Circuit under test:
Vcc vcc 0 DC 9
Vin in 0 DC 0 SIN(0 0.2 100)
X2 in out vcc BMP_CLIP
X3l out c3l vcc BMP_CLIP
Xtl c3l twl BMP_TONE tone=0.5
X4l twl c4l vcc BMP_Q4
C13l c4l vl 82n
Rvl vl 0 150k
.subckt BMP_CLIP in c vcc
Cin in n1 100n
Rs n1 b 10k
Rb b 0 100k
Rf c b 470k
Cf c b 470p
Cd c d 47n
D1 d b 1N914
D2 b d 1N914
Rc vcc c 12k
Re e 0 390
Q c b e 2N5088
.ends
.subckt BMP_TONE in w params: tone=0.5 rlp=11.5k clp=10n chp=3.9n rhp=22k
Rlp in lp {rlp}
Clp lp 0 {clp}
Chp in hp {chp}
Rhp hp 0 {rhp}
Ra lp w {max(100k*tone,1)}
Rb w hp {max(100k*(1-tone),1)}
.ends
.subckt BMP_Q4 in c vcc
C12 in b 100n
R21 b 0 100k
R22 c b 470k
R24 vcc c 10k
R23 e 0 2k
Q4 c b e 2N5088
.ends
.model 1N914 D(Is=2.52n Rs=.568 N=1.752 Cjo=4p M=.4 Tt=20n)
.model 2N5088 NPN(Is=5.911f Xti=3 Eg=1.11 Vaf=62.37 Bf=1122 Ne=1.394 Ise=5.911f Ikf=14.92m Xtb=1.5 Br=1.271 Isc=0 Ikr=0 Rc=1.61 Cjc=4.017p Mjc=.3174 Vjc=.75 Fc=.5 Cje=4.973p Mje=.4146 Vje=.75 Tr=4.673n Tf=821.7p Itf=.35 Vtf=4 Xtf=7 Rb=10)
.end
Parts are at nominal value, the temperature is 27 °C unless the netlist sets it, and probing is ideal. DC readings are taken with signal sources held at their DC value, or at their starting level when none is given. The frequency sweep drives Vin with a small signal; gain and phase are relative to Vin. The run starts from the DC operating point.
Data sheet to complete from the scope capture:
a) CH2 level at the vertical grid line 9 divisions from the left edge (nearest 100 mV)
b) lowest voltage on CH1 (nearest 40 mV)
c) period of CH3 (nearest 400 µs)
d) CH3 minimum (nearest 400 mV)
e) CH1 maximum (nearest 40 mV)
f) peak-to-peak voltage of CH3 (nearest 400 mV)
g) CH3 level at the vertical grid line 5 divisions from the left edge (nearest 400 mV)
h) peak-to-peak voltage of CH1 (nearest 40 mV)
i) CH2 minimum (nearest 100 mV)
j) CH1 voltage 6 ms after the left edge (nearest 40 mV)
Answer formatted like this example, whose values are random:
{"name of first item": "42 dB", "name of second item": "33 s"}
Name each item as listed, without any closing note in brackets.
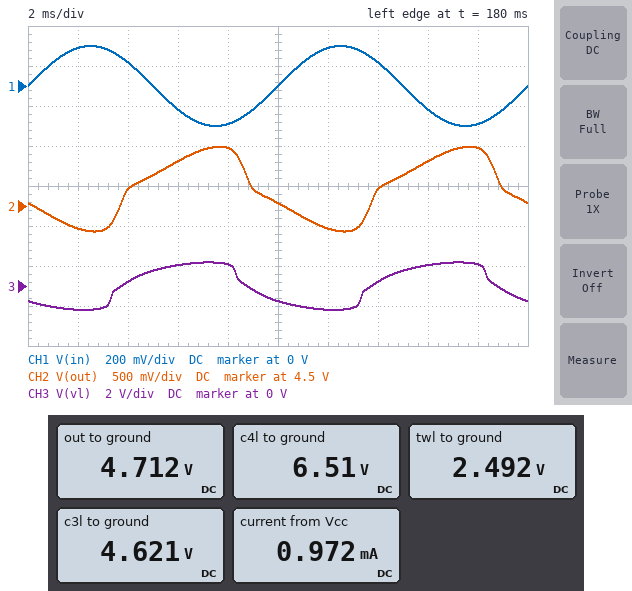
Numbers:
{"CH2 level at the vertical grid line 9 divisions from the left edge": "5.2 V", "lowest voltage on CH1": "-200 mV", "period of CH3": "10.0 ms", "CH3 minimum": "-1.2 V", "CH1 maximum": "200 mV", "peak-to-peak voltage of CH3": "2.4 V", "CH3 level at the vertical grid line 5 divisions from the left edge": "-800 mV", "peak-to-peak voltage of CH1": "400 mV", "CH2 minimum": "4.2 V", "CH1 voltage 6 ms after the left edge": "-120 mV"}
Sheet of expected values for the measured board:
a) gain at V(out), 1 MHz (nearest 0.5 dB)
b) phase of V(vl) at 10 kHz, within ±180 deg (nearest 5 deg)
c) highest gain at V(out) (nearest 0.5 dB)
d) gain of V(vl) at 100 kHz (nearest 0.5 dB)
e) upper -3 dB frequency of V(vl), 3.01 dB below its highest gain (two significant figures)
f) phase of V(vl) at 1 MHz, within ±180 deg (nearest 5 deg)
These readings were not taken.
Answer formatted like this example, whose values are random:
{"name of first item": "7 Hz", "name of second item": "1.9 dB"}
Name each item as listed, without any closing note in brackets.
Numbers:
{"gain at V(out), 1 MHz": "-26.0 dB", "phase of V(vl) at 10 kHz, within ±180 deg": "45 deg", "highest gain at V(out)": "20.5 dB", "gain of V(vl) at 100 kHz": "-18.5 dB", "upper -3 dB frequency of V(vl), 3.01 dB below its highest gain": "790 Hz", "phase of V(vl) at 1 MHz, within ±180 deg": "-165 deg"}
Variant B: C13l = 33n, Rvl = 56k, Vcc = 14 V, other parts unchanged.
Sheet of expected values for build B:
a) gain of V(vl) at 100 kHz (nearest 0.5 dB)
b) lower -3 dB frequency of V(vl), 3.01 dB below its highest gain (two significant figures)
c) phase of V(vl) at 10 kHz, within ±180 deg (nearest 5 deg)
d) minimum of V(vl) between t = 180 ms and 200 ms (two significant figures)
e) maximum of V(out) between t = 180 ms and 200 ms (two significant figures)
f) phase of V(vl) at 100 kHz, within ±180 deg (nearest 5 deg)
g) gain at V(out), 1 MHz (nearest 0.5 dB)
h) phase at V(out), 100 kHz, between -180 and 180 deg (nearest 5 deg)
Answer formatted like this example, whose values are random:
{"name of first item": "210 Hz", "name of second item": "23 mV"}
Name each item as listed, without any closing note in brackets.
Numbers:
{"gain of V(vl) at 100 kHz": "-19.0 dB", "lower -3 dB frequency of V(vl), 3.01 dB below its highest gain": "98 Hz", "phase of V(vl) at 10 kHz, within ±180 deg": "40 deg", "minimum of V(vl) between t = 180 ms and 200 ms": "-880 mV", "maximum of V(out) between t = 180 ms and 200 ms": "6.3 V", "phase of V(vl) at 100 kHz, within ±180 deg": "-15 deg", "gain at V(out), 1 MHz": "-26.5 dB", "phase at V(out), 100 kHz, between -180 and 180 deg": "85 deg"}
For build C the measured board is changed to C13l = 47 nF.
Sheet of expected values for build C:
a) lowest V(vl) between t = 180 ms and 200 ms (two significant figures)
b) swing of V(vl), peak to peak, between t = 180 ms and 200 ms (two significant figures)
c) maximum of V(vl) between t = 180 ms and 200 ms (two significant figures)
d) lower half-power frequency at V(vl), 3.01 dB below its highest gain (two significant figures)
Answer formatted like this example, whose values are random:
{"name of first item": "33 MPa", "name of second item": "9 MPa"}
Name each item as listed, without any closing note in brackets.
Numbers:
{"lowest V(vl) between t = 180 ms and 200 ms": "-1.1 V", "swing of V(vl), peak to peak, between t = 180 ms and 200 ms": "2.3 V", "maximum of V(vl) between t = 180 ms and 200 ms": "1.1 V", "lower half-power frequency at V(vl), 3.01 dB below its highest gain": "74 Hz"}
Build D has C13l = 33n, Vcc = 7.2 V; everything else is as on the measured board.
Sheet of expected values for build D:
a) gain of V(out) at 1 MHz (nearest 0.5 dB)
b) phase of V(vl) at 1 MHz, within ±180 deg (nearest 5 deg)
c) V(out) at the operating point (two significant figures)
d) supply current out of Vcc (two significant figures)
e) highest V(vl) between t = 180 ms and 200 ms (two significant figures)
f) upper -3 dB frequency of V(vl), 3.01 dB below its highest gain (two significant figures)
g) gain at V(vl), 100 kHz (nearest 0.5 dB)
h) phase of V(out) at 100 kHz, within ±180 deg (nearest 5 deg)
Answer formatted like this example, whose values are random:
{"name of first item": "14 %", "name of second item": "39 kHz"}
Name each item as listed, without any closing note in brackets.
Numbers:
{"gain of V(out) at 1 MHz": "-25.5 dB", "phase of V(vl) at 1 MHz, within ±180 deg": "-170 deg", "V(out) at the operating point": "4.3 V", "supply current out of Vcc": "660 µA", "highest V(vl) between t = 180 ms and 200 ms": "1.0 V", "upper -3 dB frequency of V(vl), 3.01 dB below its highest gain": "800 Hz", "gain at V(vl), 100 kHz": "-19.0 dB", "phase of V(out) at 100 kHz, within ±180 deg": "85 deg"}
